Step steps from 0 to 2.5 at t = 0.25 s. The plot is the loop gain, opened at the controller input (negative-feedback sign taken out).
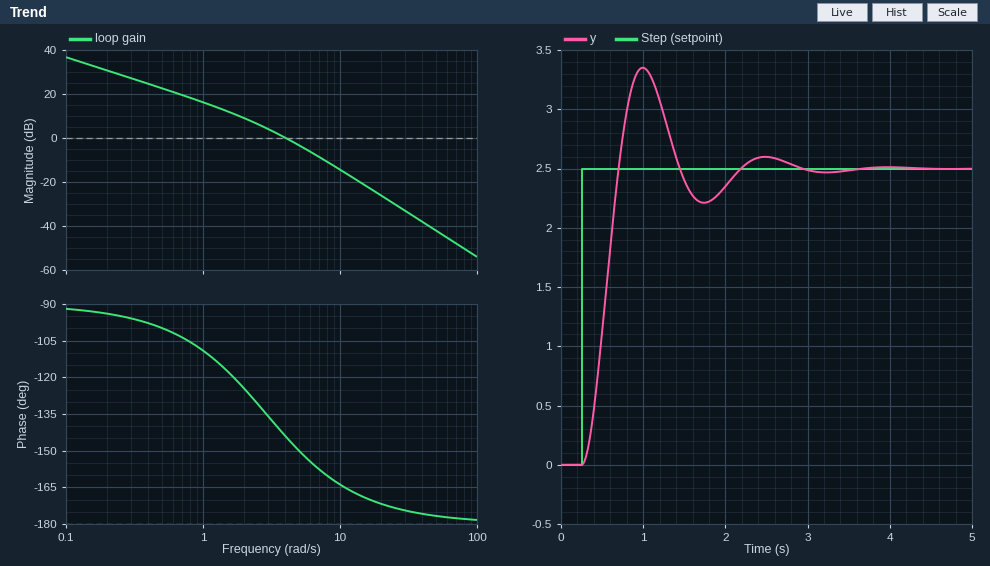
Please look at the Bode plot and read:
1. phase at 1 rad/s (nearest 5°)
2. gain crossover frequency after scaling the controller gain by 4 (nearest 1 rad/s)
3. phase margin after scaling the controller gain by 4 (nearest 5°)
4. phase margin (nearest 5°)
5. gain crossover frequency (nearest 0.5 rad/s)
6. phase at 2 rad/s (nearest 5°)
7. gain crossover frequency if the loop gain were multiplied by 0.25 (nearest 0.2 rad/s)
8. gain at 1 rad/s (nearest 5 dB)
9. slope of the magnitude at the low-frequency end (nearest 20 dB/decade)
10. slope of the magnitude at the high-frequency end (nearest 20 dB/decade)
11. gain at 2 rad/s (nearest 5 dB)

-110°
9 rad/s
20°
35°
4.0 rad/s
-125°
1.6 rad/s
15 dB
-20 dB/decade
-40 dB/decade
10 dB
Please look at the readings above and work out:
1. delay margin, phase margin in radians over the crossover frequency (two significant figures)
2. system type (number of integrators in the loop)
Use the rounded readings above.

0.15 s
1
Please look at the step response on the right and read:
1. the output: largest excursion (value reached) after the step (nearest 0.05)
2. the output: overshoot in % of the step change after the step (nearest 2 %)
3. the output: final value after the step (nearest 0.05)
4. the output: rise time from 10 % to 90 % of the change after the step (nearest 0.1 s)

3.35
34 %
2.50
0.3 s
